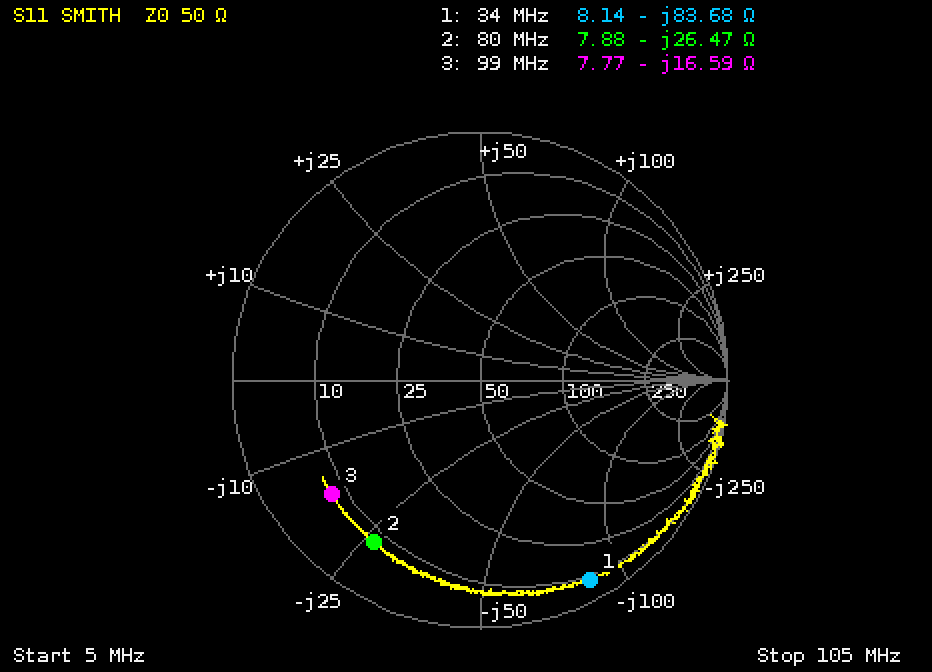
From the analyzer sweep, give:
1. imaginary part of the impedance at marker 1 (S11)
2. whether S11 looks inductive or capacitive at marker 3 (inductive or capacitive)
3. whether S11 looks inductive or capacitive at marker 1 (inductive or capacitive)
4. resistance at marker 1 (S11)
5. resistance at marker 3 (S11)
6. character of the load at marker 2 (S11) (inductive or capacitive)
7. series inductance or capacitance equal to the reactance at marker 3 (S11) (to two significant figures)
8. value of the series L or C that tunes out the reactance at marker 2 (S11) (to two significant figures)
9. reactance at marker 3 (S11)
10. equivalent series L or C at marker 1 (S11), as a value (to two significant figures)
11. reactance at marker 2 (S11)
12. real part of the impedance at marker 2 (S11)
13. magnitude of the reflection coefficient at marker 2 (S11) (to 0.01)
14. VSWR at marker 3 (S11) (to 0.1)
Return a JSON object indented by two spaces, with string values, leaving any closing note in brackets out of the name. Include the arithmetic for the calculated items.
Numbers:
{
  "imaginary part of the impedance at marker 1": "-83.68 Ω",
  "whether S11 looks inductive or capacitive at marker 3": "capacitive",
  "whether S11 looks inductive or capacitive at marker 1": "capacitive",
  "resistance at marker 1": "8.14 Ω",
  "resistance at marker 3": "7.77 Ω",
  "character of the load at marker 2 (S11)": "capacitive",
  "series inductance or capacitance equal to the reactance at marker 3 (S11)": "C = 1/(2π × 99 MHz × 16.59 Ω) ≈ 97 pF",
  "value of the series L or C that tunes out the reactance at marker 2 (S11)": "L = 26.47 Ω/(2π × 80 MHz) ≈ 53 nH",
  "reactance at marker 3": "-16.59 Ω",
  "equivalent series L or C at marker 1 (S11), as a value": "C = 1/(2π × 34 MHz × 83.68 Ω) ≈ 56 pF",
  "reactance at marker 2": "-26.47 Ω",
  "real part of the impedance at marker 2": "7.88 Ω",
  "magnitude of the reflection coefficient at marker 2 (S11)": "0.78",
  "VSWR at marker 3 (S11)": "7.2"
}
